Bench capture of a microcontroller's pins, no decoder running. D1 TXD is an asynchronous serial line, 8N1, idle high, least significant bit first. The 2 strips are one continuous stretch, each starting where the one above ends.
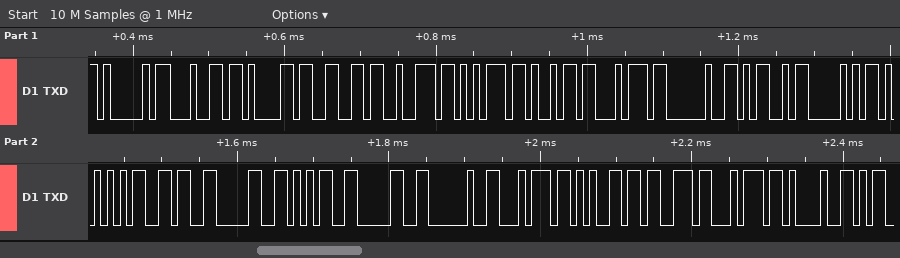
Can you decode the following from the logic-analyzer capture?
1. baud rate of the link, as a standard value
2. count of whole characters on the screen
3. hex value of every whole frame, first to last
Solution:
115200 baud
22
41 64 61 66 72 75 69 74 20 4D 50 55 36 30 35 30 20 74 65 73 74 21
